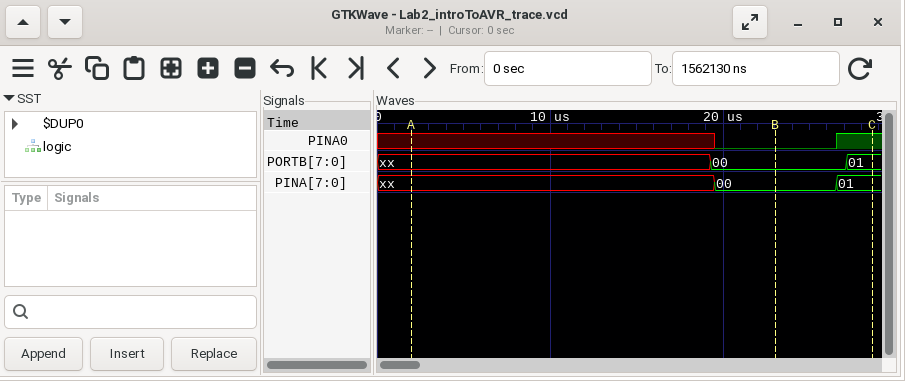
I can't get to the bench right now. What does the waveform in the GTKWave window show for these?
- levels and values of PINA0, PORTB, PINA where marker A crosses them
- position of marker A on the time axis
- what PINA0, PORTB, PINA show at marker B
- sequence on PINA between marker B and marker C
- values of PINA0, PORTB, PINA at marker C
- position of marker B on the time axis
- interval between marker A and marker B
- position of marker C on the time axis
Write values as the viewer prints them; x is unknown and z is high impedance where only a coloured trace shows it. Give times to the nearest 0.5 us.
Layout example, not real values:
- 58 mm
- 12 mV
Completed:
- PINA0=x, PORTB=xx, PINA=xx
- 2 us
- PINA0=0, PORTB=00, PINA=00
- 00, 01
- PINA0=1, PORTB=01, PINA=01
- 23 us
- 21 us
- 28.5 us
